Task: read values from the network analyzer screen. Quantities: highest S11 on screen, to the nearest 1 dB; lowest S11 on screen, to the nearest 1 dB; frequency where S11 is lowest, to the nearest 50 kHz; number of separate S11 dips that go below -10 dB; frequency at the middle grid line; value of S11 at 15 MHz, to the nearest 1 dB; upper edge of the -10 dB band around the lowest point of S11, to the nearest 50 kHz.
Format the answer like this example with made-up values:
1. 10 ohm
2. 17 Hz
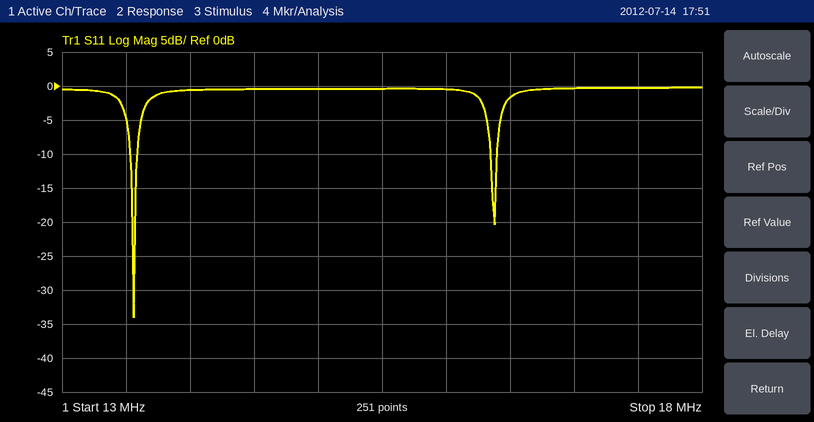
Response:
1. 0 dB
2. -34 dB
3. 13.55 MHz
4. 2
5. 15.5 MHz
6. 0 dB
7. 13.60 MHz
